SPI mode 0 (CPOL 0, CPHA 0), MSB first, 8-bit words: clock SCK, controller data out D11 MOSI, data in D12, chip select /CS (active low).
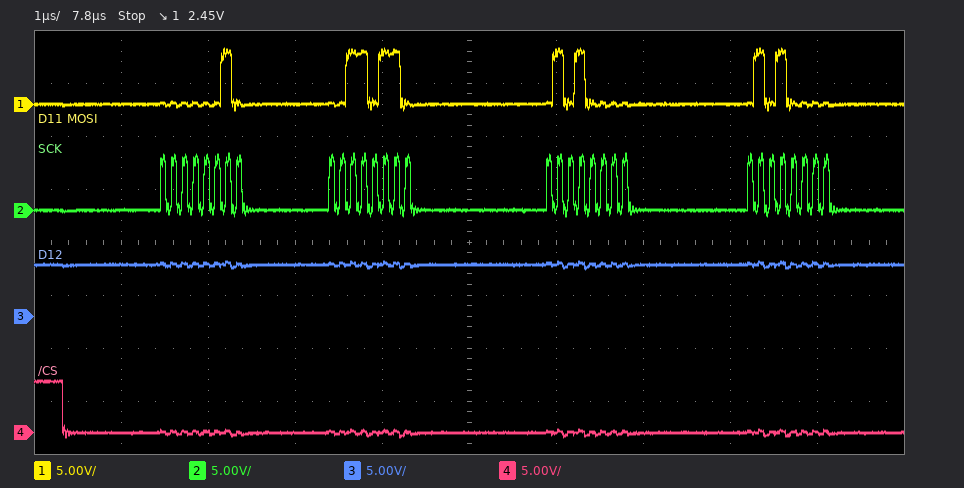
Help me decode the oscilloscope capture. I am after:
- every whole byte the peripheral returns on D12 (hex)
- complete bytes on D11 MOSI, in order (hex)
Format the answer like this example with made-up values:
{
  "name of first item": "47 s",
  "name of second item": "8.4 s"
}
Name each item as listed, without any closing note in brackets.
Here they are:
{
  "every whole byte the peripheral returns on D12": "FF FF FF FF",
  "complete bytes on D11 MOSI, in order": "02 36 50 50"
}
